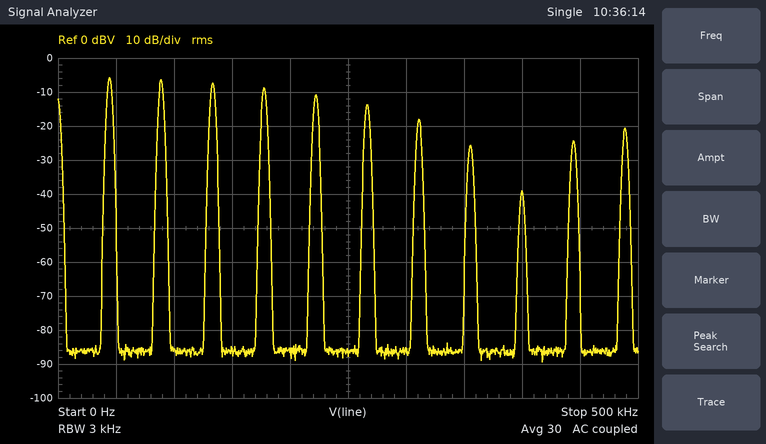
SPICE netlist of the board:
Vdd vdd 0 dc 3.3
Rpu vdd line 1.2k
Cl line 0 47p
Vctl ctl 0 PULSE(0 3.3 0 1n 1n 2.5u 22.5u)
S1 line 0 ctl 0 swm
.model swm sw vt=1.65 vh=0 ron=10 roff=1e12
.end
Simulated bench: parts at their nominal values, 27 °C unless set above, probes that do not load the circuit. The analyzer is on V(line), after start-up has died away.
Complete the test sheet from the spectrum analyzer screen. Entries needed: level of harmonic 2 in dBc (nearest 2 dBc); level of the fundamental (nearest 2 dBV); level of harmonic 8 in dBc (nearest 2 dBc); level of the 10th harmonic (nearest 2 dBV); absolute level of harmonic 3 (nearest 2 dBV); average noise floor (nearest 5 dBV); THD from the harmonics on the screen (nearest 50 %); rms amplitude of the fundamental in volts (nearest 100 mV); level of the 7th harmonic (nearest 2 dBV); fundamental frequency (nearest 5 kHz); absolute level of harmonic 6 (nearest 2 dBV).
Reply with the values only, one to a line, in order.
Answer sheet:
0 dBc
-6 dBV
-20 dBc
-24 dBV
-8 dBV
-85 dBV
150 %
500 mV
-18 dBV
45 kHz
-14 dBV
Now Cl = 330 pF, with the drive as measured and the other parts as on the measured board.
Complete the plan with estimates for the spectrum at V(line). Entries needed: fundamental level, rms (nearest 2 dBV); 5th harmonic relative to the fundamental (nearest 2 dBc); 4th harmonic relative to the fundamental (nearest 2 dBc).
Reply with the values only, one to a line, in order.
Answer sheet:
-4 dBV
-8 dBc
-4 dBc
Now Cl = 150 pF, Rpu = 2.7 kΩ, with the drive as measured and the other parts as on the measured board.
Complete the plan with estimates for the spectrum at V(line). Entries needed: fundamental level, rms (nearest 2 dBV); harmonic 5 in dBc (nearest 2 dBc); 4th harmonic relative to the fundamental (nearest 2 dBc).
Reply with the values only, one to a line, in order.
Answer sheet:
-4 dBV
-8 dBc
-4 dBc
